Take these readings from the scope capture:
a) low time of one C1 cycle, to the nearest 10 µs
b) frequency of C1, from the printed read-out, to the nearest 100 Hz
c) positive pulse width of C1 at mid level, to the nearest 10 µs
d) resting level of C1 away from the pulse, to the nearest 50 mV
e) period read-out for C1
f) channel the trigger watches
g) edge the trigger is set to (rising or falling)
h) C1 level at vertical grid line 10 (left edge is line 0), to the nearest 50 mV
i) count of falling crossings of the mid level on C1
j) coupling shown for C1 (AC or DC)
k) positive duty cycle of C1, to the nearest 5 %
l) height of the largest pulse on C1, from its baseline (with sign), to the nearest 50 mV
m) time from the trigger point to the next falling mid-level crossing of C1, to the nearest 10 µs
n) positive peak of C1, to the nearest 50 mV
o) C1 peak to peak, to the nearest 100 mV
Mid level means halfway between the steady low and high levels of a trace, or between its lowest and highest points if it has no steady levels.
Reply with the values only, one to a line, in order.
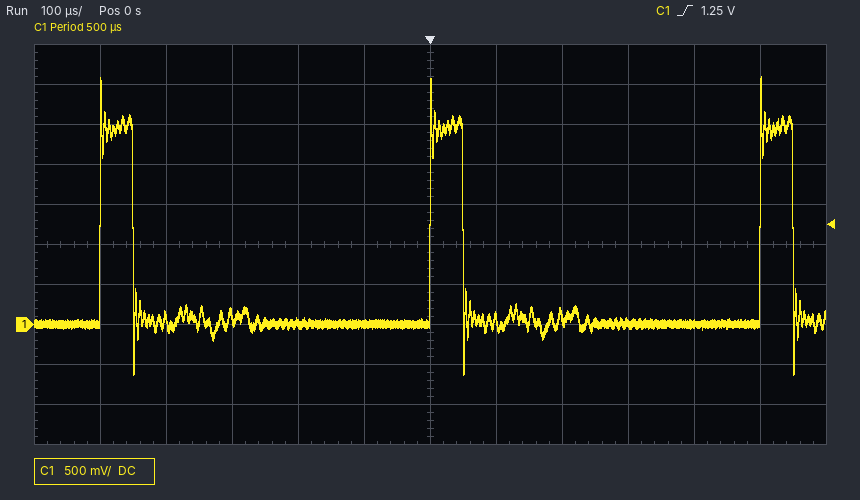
450 µs
2.0 kHz
50 µs
0 mV
500 µs
C1
rising
0 mV
3
DC
10 %
+3.10 V
50 µs
3.10 V
3.70 V
